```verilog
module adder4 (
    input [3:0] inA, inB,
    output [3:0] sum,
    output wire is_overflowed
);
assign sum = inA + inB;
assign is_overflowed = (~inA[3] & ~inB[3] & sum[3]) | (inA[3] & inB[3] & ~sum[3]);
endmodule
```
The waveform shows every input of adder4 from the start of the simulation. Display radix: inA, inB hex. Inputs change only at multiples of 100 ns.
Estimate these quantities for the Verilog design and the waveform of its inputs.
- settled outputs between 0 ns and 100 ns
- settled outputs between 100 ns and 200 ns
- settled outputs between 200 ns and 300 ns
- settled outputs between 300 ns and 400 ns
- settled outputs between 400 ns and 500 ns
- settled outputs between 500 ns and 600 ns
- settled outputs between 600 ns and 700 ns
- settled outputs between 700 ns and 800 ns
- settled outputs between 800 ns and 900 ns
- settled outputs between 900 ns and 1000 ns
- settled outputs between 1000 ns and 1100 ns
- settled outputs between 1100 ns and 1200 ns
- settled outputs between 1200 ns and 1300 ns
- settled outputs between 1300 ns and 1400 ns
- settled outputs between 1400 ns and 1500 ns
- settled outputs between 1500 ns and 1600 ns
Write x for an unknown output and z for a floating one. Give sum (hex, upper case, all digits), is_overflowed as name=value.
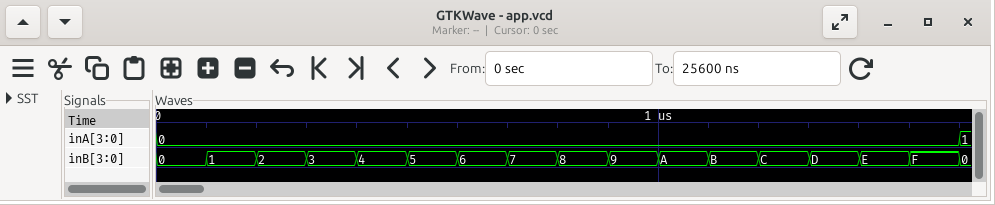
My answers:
sum=0, is_overflowed=0
sum=1, is_overflowed=0
sum=2, is_overflowed=0
sum=3, is_overflowed=0
sum=4, is_overflowed=0
sum=5, is_overflowed=0
sum=6, is_overflowed=0
sum=7, is_overflowed=0
sum=8, is_overflowed=0
sum=9, is_overflowed=0
sum=A, is_overflowed=0
sum=B, is_overflowed=0
sum=C, is_overflowed=0
sum=D, is_overflowed=0
sum=E, is_overflowed=0
sum=F, is_overflowed=0
